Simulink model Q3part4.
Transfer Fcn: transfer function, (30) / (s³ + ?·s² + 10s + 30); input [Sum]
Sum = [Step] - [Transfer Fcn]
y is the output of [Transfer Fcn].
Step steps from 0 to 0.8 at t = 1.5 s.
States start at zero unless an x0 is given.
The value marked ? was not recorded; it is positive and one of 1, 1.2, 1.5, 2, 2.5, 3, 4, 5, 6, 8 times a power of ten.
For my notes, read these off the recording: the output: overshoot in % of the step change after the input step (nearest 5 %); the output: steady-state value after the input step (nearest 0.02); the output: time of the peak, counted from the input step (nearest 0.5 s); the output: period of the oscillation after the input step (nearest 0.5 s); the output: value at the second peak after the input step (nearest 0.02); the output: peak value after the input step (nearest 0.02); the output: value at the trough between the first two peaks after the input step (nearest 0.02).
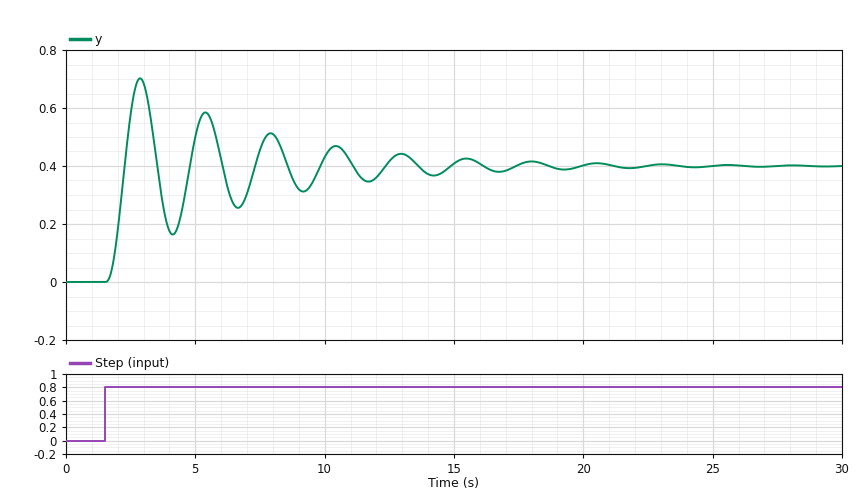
75 %
0.40
1.5 s
2.5 s
0.58
0.70
0.16
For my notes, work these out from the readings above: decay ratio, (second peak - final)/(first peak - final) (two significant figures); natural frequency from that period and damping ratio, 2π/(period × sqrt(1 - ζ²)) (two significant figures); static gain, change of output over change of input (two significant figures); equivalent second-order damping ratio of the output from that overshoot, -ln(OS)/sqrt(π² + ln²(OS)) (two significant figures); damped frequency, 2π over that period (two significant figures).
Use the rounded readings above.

0.60
2.5 rad/s
0.50
0.091
2.5 rad/s
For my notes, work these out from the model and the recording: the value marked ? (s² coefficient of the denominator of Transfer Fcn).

10
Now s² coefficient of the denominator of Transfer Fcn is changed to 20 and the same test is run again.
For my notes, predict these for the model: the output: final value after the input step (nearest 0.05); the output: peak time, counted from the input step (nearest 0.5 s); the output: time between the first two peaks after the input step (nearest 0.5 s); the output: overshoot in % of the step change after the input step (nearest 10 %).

0.40
2.0 s
3.5 s
70 %
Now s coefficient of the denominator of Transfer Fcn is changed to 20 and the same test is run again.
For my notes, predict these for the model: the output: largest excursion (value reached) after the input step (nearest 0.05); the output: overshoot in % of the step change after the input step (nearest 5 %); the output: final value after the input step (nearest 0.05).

0.55
35 %
0.40
